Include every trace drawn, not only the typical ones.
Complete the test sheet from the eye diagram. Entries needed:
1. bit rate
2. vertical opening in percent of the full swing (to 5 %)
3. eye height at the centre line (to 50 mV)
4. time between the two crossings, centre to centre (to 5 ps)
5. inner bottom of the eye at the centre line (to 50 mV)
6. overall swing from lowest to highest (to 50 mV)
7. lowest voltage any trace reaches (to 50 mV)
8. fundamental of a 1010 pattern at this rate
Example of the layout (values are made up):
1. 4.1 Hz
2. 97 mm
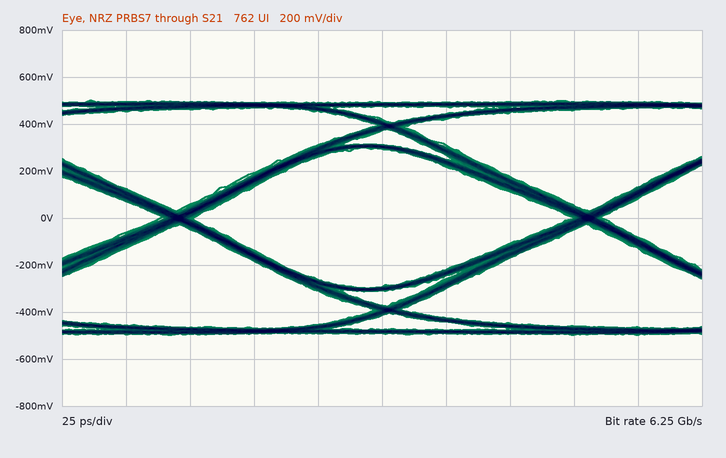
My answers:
1. 6.25 Gb/s
2. 60 %
3. 600 mV
4. 160 ps
5. -300 mV
6. 1.00 V
7. -500 mV
8. 3.125 GHz
